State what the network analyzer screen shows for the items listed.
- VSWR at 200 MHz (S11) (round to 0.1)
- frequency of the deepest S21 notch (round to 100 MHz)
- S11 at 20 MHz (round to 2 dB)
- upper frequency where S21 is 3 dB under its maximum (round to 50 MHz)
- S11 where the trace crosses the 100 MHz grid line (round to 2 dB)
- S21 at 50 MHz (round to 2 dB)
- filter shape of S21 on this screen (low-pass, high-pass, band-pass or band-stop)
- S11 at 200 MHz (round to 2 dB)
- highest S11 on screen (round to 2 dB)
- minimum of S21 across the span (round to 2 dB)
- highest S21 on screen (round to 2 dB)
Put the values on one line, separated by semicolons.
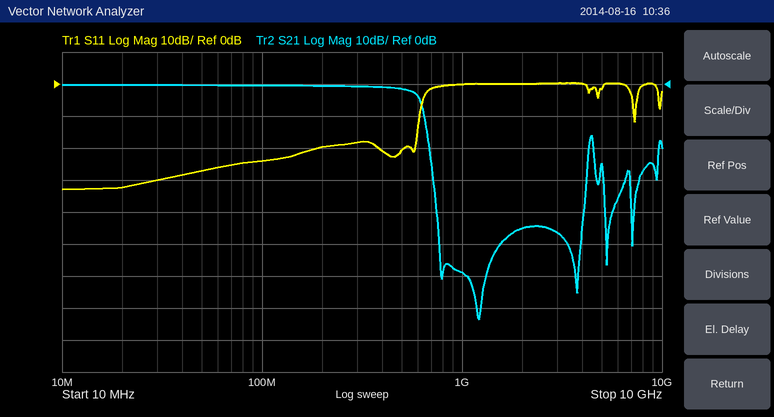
1.2; 1.2 GHz; -32 dB; 600 MHz; -24 dB; 0 dB; low-pass; -20 dB; 0 dB; -74 dB; 0 dB
